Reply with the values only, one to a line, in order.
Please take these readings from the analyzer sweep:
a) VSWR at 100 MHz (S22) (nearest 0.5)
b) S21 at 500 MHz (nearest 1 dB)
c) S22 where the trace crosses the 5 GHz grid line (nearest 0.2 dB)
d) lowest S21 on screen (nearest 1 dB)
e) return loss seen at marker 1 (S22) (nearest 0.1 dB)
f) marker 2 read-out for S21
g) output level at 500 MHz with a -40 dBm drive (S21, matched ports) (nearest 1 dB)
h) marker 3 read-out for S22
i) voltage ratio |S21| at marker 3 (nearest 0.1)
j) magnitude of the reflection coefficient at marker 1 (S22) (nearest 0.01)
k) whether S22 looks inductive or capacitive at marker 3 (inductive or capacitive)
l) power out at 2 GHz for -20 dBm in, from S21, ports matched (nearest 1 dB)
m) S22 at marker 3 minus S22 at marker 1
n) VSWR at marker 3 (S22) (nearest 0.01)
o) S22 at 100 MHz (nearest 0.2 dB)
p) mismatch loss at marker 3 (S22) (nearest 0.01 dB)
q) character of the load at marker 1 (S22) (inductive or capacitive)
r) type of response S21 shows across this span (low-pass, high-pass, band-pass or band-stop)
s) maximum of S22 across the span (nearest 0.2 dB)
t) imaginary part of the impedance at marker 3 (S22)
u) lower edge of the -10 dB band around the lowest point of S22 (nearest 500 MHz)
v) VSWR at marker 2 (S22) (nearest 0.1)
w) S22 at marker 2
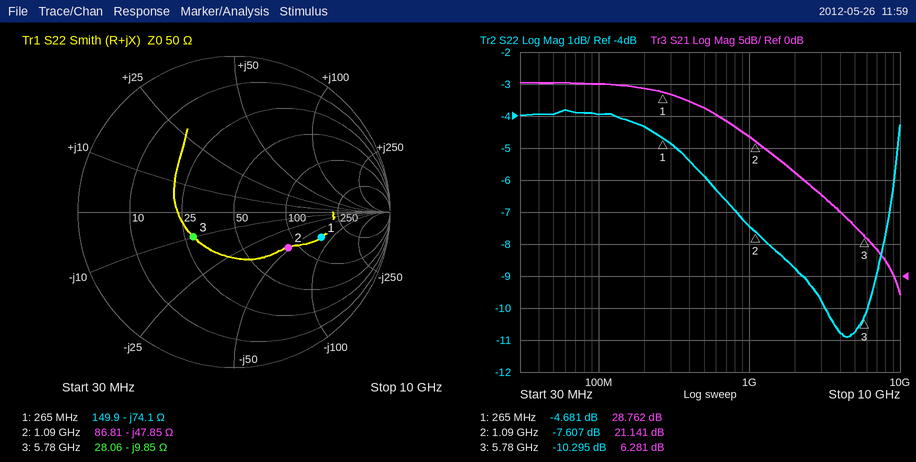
4.5
26 dB
-10.8 dB
-3 dB
4.7 dB
21.141 dB
-14 dBm
-10.295 dB
2.1
0.58
capacitive
-4 dBm
-5.614 dB
1.88
-4.0 dB
0.43 dB
capacitive
low-pass
-3.8 dB
-9.85 Ω
3.0 GHz
2.4
-7.607 dB
